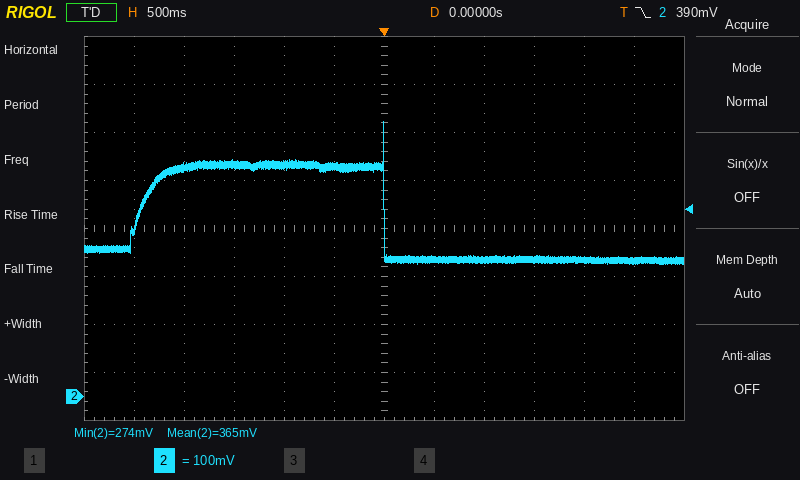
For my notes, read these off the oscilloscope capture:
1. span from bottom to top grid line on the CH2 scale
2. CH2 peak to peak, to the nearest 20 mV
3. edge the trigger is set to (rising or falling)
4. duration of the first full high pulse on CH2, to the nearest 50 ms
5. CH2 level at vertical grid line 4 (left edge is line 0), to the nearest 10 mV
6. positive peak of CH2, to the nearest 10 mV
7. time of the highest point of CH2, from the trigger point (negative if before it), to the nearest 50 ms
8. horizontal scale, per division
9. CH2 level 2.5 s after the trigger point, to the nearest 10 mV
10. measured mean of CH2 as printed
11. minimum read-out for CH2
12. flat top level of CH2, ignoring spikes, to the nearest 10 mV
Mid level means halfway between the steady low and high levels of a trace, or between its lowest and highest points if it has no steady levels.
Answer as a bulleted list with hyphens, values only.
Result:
- 800 mV
- 300 mV
- falling
- 2.45 s
- 480 mV
- 570 mV
- 0 ms
- 500 ms
- 280 mV
- 365 mV
- 274 mV
- 480 mV
